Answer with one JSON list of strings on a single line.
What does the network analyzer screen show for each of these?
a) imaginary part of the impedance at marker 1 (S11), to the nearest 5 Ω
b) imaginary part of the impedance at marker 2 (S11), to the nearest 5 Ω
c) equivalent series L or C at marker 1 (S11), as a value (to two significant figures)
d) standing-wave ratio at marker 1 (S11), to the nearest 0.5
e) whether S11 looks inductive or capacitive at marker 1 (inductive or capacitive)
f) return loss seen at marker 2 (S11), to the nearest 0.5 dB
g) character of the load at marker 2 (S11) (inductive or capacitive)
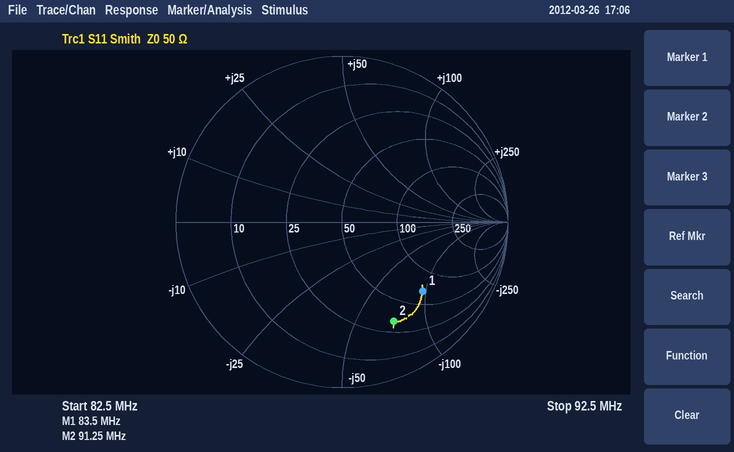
["-95 Ω", "-70 Ω", "20 pF", "4.5", "capacitive", "3.5 dB", "capacitive"]
